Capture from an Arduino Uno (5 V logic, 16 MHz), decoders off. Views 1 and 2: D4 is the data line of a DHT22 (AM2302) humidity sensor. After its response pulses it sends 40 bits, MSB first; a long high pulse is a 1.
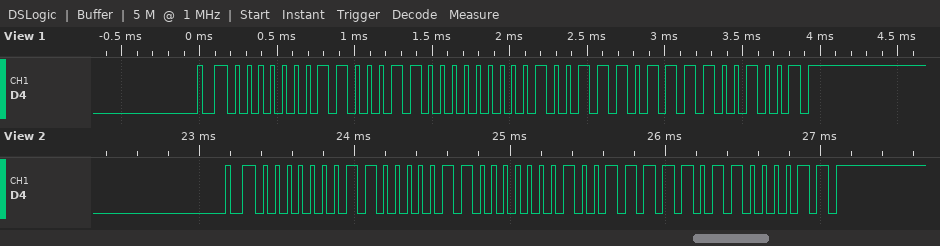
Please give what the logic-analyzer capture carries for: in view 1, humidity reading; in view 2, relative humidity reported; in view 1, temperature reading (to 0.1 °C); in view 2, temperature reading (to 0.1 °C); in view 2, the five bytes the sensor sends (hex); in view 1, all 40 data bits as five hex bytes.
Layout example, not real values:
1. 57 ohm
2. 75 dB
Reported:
1. 39.6 %
2. 38.7 %
3. 31.5 °C
4. 31.8 °C
5. 01 83 01 3E C3
6. 01 8C 01 3B C9
